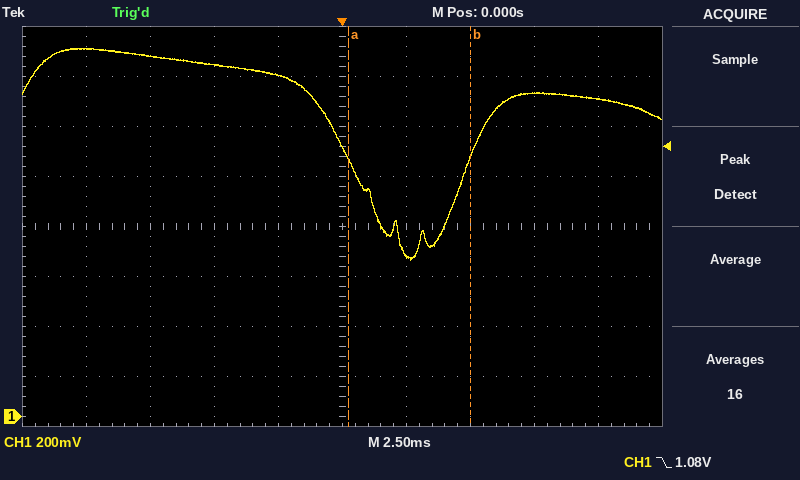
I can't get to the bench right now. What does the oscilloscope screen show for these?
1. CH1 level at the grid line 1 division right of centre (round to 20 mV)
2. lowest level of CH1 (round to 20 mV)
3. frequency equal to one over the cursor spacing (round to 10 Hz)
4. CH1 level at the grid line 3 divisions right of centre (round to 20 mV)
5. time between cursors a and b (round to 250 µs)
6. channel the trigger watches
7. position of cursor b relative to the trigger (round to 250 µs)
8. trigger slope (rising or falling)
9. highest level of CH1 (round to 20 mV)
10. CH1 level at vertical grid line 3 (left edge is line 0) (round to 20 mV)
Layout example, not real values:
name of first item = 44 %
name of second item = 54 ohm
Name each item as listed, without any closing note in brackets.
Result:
CH1 level at the grid line 1 division right of centre = 640 mV
lowest level of CH1 = 620 mV
frequency equal to one over the cursor spacing = 210 Hz
CH1 level at the grid line 3 divisions right of centre = 1.30 V
time between cursors a and b = 4.75 ms
channel the trigger watches = CH1
position of cursor b relative to the trigger = +5.00 ms
trigger slope = falling
highest level of CH1 = 1.48 V
CH1 level at vertical grid line 3 (left edge is line 0) = 1.40 V
